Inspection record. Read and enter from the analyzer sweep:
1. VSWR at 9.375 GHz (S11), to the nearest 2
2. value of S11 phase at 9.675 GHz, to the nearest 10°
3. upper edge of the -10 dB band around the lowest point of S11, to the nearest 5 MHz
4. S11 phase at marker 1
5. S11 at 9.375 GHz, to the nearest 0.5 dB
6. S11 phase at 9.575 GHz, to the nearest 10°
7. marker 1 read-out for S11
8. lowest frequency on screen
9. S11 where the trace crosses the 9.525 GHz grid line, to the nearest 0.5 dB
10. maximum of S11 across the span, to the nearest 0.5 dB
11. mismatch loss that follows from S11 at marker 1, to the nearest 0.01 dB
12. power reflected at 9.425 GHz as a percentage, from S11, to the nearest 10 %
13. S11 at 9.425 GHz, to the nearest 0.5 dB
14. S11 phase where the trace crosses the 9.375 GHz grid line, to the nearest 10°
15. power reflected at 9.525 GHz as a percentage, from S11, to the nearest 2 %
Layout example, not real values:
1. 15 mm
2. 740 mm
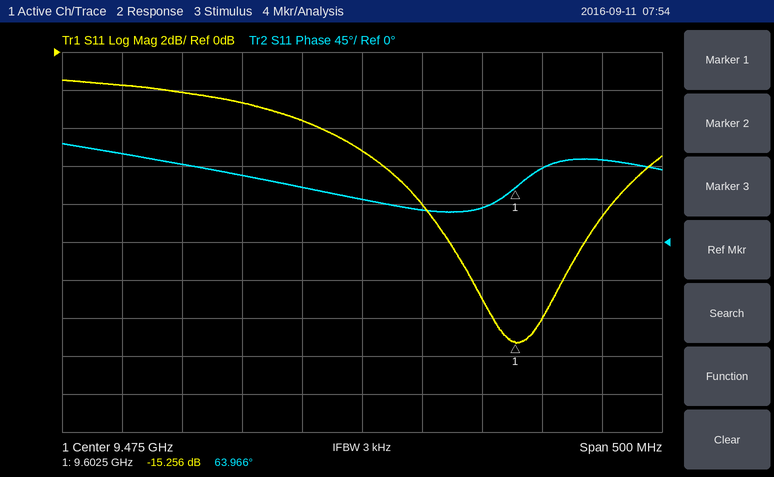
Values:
1. 6
2. 100°
3. 9.660 GHz
4. 63.966°
5. -2.5 dB
6. 40°
7. -15.256 dB
8. 9.225 GHz
9. -8.0 dB
10. -1.5 dB
11. 0.13 dB
12. 40 %
13. -3.5 dB
14. 80°
15. 16 %
